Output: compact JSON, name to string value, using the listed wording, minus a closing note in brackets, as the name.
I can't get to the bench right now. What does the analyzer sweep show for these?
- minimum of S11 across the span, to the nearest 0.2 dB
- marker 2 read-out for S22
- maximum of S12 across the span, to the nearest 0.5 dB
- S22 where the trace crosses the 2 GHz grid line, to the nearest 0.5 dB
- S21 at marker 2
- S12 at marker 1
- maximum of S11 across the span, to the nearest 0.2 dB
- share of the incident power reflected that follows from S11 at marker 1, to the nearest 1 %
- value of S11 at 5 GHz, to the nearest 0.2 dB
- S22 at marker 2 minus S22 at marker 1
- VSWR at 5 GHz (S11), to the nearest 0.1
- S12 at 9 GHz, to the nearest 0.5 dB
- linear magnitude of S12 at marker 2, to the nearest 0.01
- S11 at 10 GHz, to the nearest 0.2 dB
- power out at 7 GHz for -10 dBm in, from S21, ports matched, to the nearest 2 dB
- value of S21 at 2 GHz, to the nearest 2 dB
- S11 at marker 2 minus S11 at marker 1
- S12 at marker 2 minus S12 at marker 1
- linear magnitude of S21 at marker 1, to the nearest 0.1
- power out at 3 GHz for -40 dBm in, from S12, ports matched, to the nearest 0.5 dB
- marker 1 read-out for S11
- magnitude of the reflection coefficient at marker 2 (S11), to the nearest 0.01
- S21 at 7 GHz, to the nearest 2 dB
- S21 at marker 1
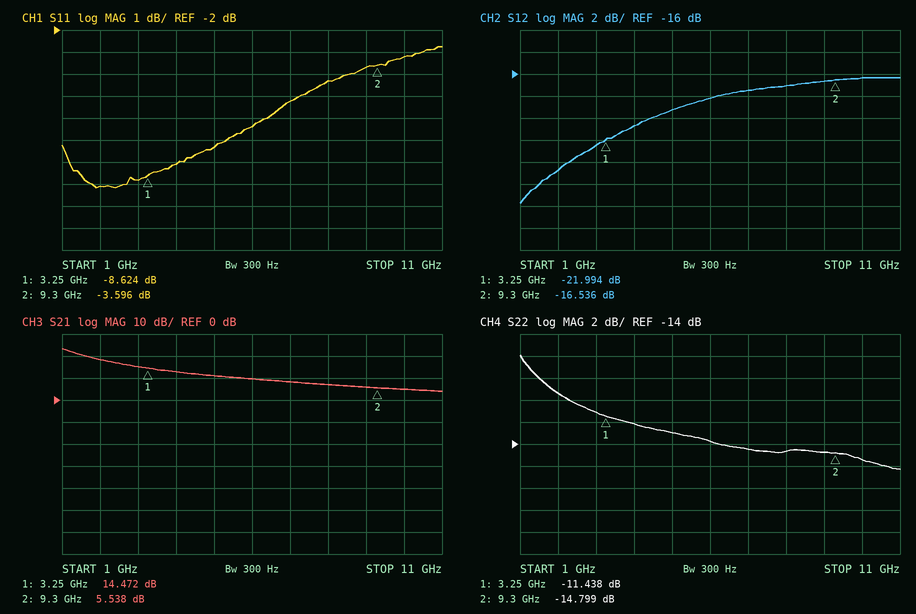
{"minimum of S11 across the span, to the nearest 0.2 dB": "-9.2 dB", "marker 2 read-out for S22": "-14.799 dB", "maximum of S12 across the span, to the nearest 0.5 dB": "-16.5 dB", "S22 where the trace crosses the 2 GHz grid line, to the nearest 0.5 dB": "-9.5 dB", "S21 at marker 2": "5.538 dB", "S12 at marker 1": "-21.994 dB", "maximum of S11 across the span, to the nearest 0.2 dB": "-2.8 dB", "share of the incident power reflected that follows from S11 at marker 1, to the nearest 1 %": "14 %", "value of S11 at 5 GHz, to the nearest 0.2 dB": "-7.4 dB", "S22 at marker 2 minus S22 at marker 1": "-3.361 dB", "VSWR at 5 GHz (S11), to the nearest 0.1": "2.5", "S12 at 9 GHz, to the nearest 0.5 dB": "-16.5 dB", "linear magnitude of S12 at marker 2, to the nearest 0.01": "0.15", "S11 at 10 GHz, to the nearest 0.2 dB": "-3.2 dB", "power out at 7 GHz for -10 dBm in, from S21, ports matched, to the nearest 2 dB": "-2 dBm", "value of S21 at 2 GHz, to the nearest 2 dB": "18 dB", "S11 at marker 2 minus S11 at marker 1": "5.028 dB", "S12 at marker 2 minus S12 at marker 1": "5.458 dB", "linear magnitude of S21 at marker 1, to the nearest 0.1": "5.3", "power out at 3 GHz for -40 dBm in, from S12, ports matched, to the nearest 0.5 dB": "-62.5 dBm", "marker 1 read-out for S11": "-8.624 dB", "magnitude of the reflection coefficient at marker 2 (S11), to the nearest 0.01": "0.66", "S21 at 7 GHz, to the nearest 2 dB": "8 dB", "S21 at marker 1": "14.472 dB"}
